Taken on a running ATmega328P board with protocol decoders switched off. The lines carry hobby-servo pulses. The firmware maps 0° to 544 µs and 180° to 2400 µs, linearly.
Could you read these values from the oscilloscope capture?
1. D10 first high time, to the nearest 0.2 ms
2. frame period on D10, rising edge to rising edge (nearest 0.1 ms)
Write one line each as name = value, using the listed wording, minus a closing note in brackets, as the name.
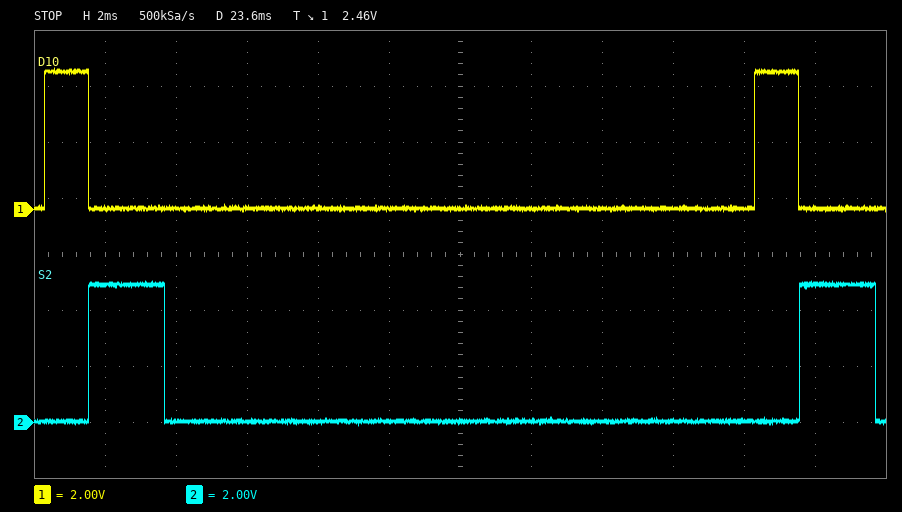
D10 first high time, to the nearest 0.2 ms = 1.2 ms
frame period on D10, rising edge to rising edge = 20.0 ms
